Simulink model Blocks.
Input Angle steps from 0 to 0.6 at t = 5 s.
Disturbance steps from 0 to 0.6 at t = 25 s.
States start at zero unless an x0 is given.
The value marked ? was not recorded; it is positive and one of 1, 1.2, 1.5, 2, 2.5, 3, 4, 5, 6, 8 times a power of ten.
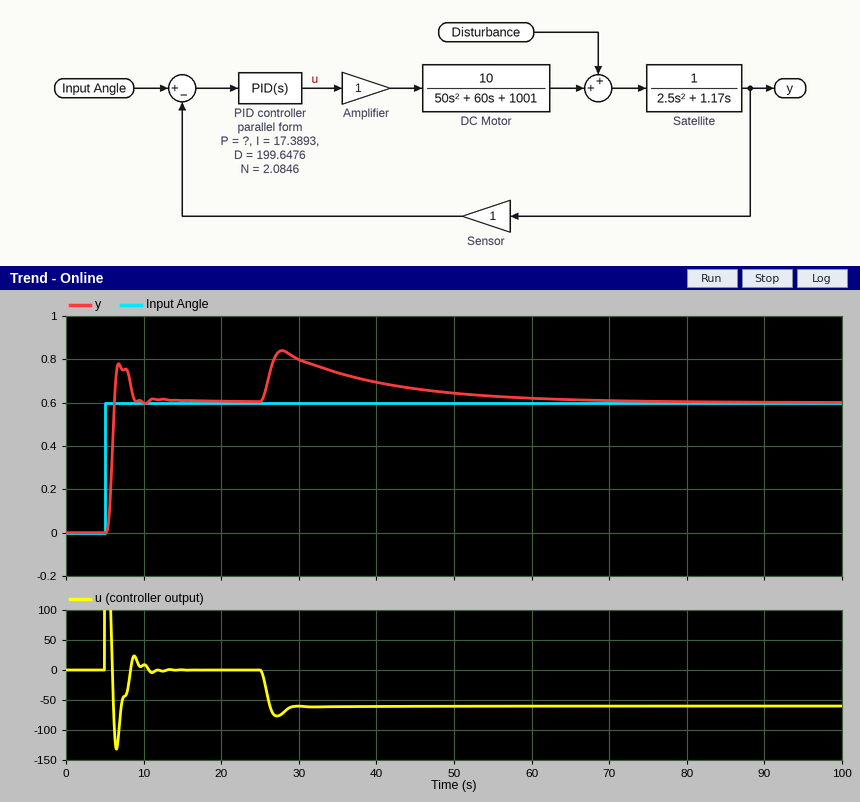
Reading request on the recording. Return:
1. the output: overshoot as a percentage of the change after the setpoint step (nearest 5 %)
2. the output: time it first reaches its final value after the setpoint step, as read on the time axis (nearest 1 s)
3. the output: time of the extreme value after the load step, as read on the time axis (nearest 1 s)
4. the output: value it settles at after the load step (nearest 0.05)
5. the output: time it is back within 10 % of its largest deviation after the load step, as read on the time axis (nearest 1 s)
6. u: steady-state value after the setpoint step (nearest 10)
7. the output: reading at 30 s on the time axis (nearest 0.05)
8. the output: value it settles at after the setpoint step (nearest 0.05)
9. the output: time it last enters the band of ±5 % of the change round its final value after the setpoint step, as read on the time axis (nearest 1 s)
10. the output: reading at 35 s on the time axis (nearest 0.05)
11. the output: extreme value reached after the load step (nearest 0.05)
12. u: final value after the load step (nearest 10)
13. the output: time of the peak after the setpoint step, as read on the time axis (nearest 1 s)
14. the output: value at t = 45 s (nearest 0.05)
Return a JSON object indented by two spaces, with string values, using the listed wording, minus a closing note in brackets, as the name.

{
  "the output: overshoot as a percentage of the change after the setpoint step": "30 %",
  "the output: time it first reaches its final value after the setpoint step, as read on the time axis": "6 s",
  "the output: time of the extreme value after the load step, as read on the time axis": "28 s",
  "the output: value it settles at after the load step": "0.60",
  "the output: time it is back within 10 % of its largest deviation after the load step, as read on the time axis": "58 s",
  "u: steady-state value after the setpoint step": "0",
  "the output: reading at 30 s on the time axis": "0.80",
  "the output: value it settles at after the setpoint step": "0.60",
  "the output: time it last enters the band of ±5 % of the change round its final value after the setpoint step, as read on the time axis": "9 s",
  "the output: reading at 35 s on the time axis": "0.75",
  "the output: extreme value reached after the load step": "0.85",
  "u: final value after the load step": "-60",
  "the output: time of the peak after the setpoint step, as read on the time axis": "7 s",
  "the output: value at t = 45 s": "0.65"
}
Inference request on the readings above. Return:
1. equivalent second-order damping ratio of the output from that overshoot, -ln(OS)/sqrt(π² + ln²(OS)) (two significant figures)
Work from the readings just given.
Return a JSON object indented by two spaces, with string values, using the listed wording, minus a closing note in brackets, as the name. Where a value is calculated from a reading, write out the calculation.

{
  "equivalent second-order damping ratio of the output from that overshoot, -ln(OS)/sqrt(π² + ln²(OS))": "ln(0.3) = -1.204; 1.204 / sqrt(9.870 + 1.450) = 0.36"
}
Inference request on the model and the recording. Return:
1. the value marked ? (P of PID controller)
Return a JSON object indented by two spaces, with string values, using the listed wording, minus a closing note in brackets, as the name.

{
  "the value marked ?": "250"
}
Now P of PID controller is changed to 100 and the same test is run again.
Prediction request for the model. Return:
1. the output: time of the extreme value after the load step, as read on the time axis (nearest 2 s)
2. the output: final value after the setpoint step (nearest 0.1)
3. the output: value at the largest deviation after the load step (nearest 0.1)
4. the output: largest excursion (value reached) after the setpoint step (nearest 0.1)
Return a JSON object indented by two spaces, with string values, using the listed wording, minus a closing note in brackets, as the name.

{
  "the output: time of the extreme value after the load step, as read on the time axis": "30 s",
  "the output: final value after the setpoint step": "0.6",
  "the output: value at the largest deviation after the load step": "1.0",
  "the output: largest excursion (value reached) after the setpoint step": "0.7"
}
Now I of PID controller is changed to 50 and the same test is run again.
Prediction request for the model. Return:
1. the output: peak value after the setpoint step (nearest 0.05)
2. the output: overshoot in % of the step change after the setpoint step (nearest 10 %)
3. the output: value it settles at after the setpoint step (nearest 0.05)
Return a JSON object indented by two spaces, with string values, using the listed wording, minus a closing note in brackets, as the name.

{
  "the output: peak value after the setpoint step": "0.80",
  "the output: overshoot in % of the step change after the setpoint step": "40 %",
  "the output: value it settles at after the setpoint step": "0.60"
}
